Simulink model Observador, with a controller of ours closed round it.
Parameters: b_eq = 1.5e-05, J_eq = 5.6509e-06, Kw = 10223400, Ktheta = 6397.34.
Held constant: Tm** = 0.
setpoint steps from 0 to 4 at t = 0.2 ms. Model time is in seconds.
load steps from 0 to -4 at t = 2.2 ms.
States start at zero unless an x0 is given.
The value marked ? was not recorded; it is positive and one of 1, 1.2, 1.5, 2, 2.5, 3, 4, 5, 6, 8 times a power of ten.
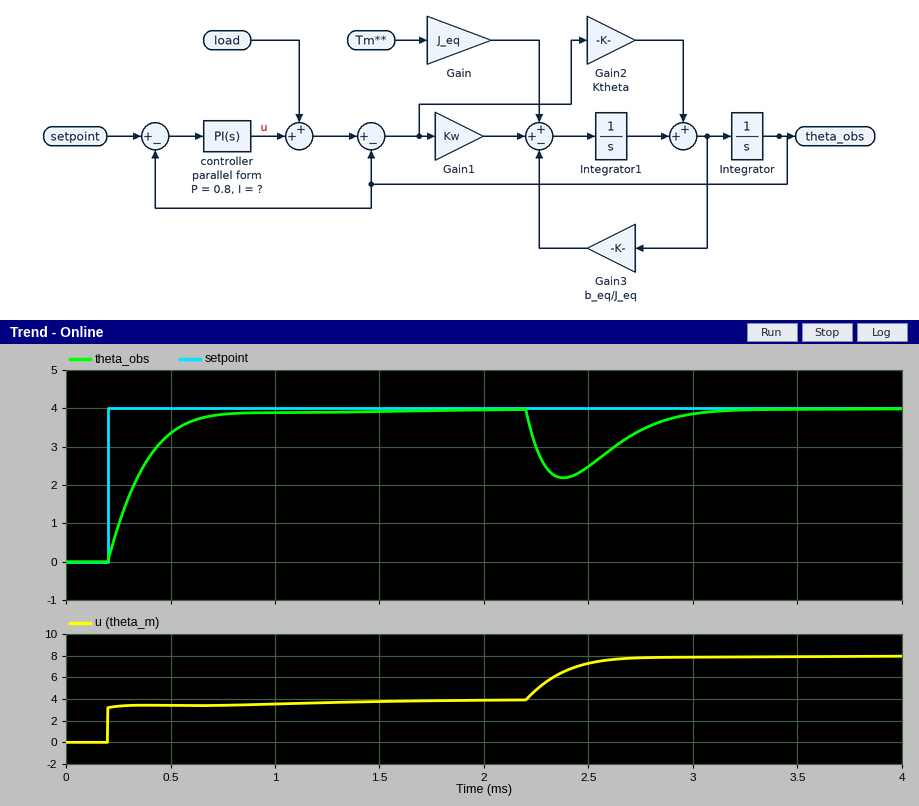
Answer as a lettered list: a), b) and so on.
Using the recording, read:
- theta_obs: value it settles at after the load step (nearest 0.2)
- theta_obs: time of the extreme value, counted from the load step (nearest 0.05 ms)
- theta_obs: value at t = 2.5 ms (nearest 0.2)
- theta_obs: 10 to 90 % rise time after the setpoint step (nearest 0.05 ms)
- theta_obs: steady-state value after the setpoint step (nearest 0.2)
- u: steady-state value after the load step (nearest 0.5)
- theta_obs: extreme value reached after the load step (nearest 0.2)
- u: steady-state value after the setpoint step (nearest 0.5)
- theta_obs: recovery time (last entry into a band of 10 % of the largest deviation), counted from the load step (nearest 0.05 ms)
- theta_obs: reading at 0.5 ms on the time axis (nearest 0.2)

a) 4.0
b) 0.20 ms
c) 2.4
d) 0.35 ms
e) 4.0
f) 8.0
g) 2.2
h) 4.0
i) 0.75 ms
j) 3.4
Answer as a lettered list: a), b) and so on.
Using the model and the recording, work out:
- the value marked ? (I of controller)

a) 5000
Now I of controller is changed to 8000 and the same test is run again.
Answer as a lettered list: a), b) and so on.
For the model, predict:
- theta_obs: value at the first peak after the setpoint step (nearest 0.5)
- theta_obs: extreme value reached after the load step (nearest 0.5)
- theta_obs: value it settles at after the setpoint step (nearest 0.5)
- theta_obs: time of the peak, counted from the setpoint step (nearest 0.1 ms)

a) 4.0
b) 2.5
c) 4.0
d) 0.4 ms
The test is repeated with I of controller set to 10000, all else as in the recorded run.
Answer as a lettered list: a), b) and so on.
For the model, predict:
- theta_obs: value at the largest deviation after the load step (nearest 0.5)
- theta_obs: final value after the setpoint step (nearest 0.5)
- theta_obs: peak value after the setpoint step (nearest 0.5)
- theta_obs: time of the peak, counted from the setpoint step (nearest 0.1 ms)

a) 2.5
b) 4.0
c) 4.5
d) 0.4 ms
